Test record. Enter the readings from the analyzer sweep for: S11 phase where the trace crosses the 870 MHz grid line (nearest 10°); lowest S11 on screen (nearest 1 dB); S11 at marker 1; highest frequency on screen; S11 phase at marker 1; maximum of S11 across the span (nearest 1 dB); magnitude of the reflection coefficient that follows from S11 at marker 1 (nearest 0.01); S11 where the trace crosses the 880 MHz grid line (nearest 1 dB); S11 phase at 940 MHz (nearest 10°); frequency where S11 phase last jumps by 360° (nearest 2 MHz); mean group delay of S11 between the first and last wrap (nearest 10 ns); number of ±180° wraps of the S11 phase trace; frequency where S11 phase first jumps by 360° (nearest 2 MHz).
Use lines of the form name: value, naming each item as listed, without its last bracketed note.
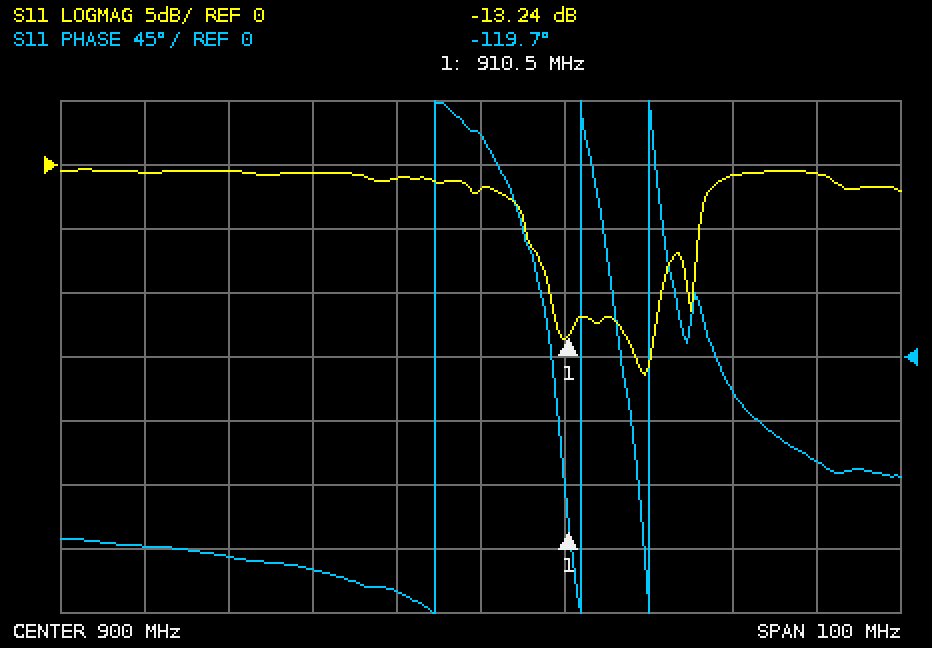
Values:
S11 phase where the trace crosses the 870 MHz grid line: -140°
lowest S11 on screen: -16 dB
S11 at marker 1: -13.24 dB
highest frequency on screen: 950 MHz
S11 phase at marker 1: -119.7°
maximum of S11 across the span: 0 dB
magnitude of the reflection coefficient that follows from S11 at marker 1: 0.22
S11 where the trace crosses the 880 MHz grid line: -1 dB
S11 phase at 940 MHz: -70°
frequency where S11 phase last jumps by 360°: 920 MHz
mean group delay of S11 between the first and last wrap: 80 ns
number of ±180° wraps of the S11 phase trace: 3
frequency where S11 phase first jumps by 360°: 894 MHz
